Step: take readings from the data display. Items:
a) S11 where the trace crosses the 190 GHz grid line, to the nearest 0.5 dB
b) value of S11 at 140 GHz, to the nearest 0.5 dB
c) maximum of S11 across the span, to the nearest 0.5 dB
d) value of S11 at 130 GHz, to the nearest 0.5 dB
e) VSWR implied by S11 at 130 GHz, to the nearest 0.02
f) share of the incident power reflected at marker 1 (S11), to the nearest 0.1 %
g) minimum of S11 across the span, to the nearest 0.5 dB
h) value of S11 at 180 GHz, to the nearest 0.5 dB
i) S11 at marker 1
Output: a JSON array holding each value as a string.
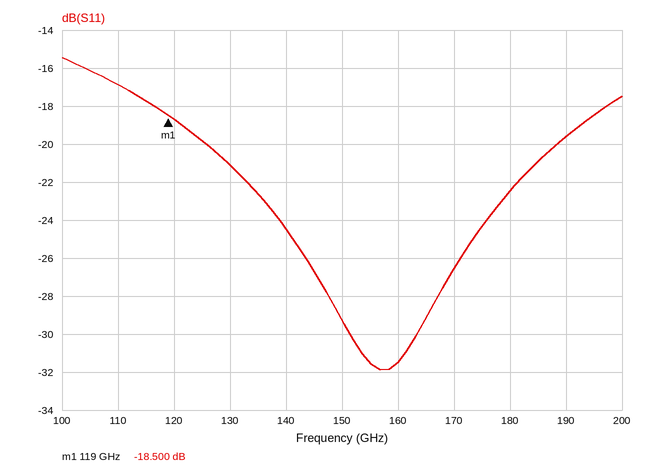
["-19.5 dB", "-24.5 dB", "-15.5 dB", "-21.0 dB", "1.20", "1.4 %", "-32.0 dB", "-22.5 dB", "-18.500 dB"]
